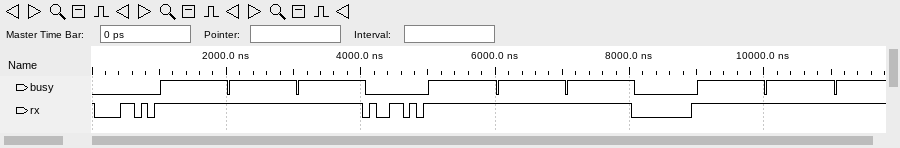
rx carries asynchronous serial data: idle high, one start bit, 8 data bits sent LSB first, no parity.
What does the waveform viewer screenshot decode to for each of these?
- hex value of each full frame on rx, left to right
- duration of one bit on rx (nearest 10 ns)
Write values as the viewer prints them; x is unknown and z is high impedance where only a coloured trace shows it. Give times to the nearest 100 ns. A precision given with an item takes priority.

58, 59, 00
100 ns
